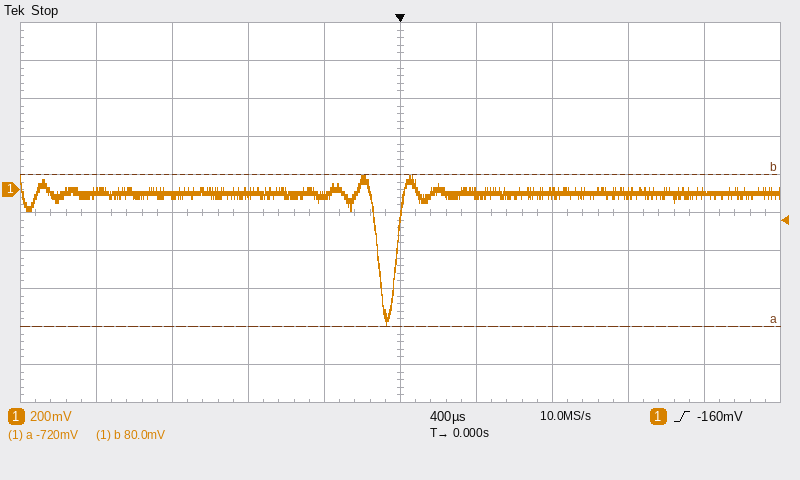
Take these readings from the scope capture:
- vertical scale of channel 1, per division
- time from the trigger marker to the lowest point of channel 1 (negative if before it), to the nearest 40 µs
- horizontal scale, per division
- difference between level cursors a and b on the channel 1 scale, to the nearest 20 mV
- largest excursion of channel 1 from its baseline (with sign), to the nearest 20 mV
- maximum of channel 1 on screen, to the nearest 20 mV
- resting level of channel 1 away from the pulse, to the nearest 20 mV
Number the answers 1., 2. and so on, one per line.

1. 200 mV
2. -80 µs
3. 400 µs
4. 800 mV
5. -700 mV
6. 80 mV
7. -20 mV
